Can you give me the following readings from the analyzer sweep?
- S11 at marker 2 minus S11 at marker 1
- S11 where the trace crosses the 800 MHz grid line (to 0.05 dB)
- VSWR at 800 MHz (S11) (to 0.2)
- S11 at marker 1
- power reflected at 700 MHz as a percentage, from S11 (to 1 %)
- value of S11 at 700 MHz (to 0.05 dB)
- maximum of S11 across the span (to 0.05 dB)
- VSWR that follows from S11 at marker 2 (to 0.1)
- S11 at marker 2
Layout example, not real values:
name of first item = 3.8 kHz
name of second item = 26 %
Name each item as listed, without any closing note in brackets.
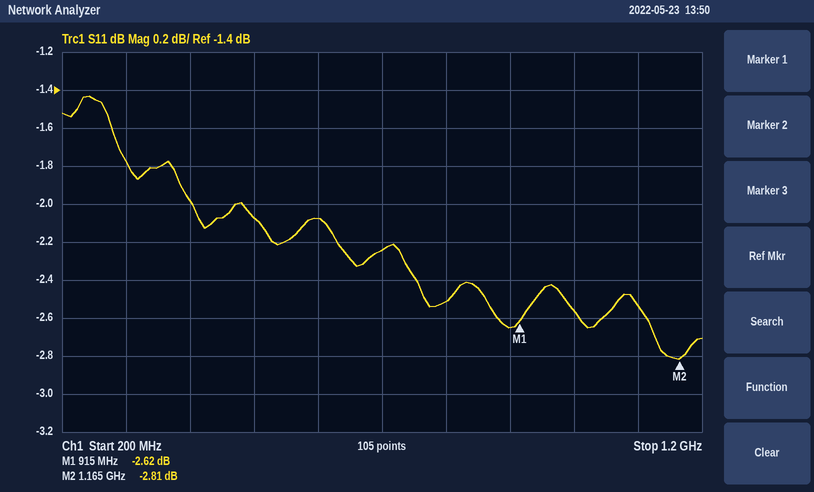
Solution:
S11 at marker 2 minus S11 at marker 1 = -0.19 dB
S11 where the trace crosses the 800 MHz grid line = -2.50 dB
VSWR at 800 MHz (S11) = 7.0
S11 at marker 1 = -2.62 dB
power reflected at 700 MHz as a percentage, from S11 = 60 %
value of S11 at 700 MHz = -2.25 dB
maximum of S11 across the span = -1.45 dB
VSWR that follows from S11 at marker 2 = 6.2
S11 at marker 2 = -2.81 dB
